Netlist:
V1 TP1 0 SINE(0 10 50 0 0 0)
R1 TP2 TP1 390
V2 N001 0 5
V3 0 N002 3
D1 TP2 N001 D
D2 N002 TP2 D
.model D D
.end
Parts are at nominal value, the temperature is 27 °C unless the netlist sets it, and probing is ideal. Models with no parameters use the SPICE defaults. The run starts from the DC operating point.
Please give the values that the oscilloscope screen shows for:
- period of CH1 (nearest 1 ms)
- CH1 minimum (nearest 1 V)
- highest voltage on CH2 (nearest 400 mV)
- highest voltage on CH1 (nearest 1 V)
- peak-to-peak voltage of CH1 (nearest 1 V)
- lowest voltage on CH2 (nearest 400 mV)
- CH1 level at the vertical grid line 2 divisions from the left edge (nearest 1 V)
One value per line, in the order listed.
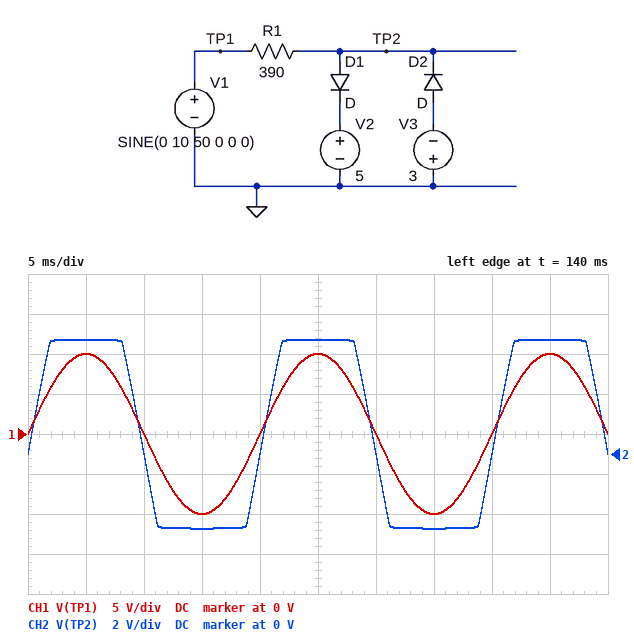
20 ms
-10 V
5.6 V
10 V
20 V
-3.6 V
0 V
